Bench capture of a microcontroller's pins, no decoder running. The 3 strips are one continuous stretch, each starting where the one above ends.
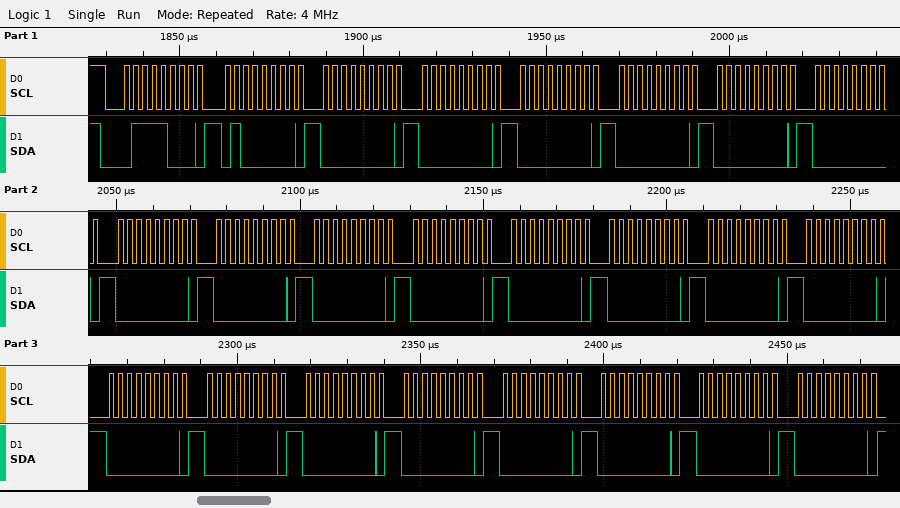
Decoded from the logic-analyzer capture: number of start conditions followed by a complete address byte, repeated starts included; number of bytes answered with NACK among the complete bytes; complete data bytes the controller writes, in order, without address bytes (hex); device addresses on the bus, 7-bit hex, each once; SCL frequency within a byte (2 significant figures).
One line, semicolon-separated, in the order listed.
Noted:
1; 0; 40 00 00 00 00 00 00 00 00 00 00 00 00 00 00 00 00 00 00 00 00 00 00; 0x3C; 400 kHz
